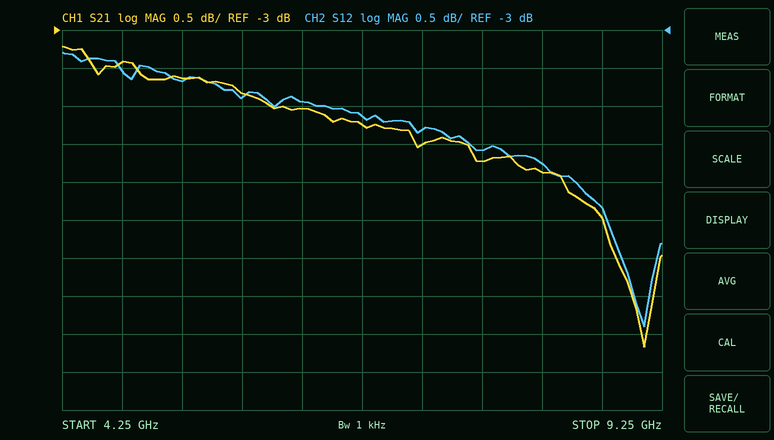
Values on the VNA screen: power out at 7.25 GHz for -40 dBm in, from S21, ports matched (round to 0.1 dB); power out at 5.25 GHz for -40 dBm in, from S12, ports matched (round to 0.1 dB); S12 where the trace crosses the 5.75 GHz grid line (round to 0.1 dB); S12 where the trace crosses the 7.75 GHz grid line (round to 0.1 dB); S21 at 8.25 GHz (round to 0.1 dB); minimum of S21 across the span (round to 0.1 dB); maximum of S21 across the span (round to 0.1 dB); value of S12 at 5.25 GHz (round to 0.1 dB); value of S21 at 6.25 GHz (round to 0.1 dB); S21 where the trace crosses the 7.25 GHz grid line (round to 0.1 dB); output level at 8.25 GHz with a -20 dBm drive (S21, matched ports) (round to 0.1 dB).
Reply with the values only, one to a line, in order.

-44.5 dBm
-43.7 dBm
-3.9 dB
-4.6 dB
-4.9 dB
-7.2 dB
-3.2 dB
-3.7 dB
-4.0 dB
-4.5 dB
-24.9 dBm
